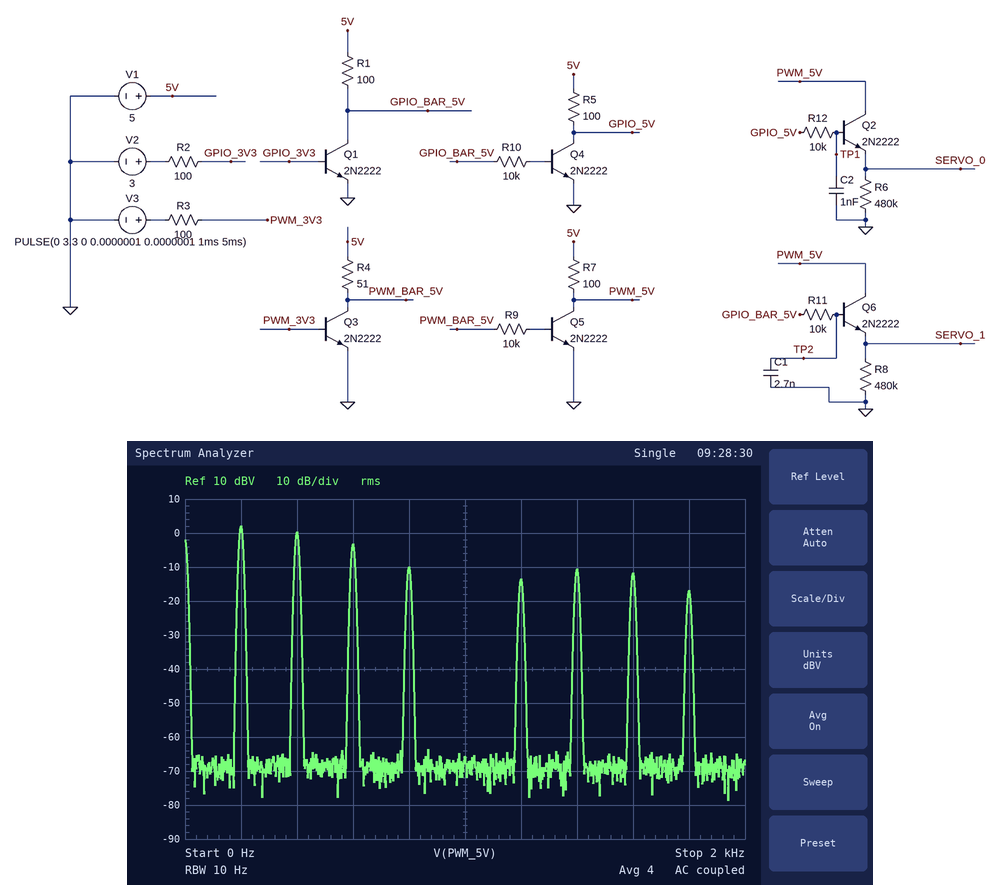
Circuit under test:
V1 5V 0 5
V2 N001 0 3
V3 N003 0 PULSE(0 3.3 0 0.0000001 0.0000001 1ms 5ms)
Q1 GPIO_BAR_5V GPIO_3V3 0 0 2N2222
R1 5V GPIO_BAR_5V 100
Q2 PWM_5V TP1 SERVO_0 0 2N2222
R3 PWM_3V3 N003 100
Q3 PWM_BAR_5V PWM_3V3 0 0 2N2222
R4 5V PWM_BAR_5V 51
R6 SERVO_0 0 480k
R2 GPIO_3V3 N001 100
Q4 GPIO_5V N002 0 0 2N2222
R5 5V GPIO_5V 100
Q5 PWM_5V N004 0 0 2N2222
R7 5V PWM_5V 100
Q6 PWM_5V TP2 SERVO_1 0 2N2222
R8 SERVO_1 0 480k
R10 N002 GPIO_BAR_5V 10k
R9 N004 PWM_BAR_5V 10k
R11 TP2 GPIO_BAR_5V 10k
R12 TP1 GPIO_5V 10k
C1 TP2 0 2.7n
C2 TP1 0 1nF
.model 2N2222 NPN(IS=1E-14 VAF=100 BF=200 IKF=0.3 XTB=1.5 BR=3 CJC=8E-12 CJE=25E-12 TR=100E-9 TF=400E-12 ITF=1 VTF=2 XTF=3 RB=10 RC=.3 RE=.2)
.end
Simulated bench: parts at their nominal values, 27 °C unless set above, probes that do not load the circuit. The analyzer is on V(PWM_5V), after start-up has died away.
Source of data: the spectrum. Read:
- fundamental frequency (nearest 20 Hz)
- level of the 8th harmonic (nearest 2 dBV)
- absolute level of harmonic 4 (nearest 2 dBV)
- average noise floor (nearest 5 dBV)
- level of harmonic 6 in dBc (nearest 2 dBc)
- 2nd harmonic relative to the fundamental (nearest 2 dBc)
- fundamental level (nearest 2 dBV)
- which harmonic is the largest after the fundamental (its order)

200 Hz
-12 dBV
-10 dBV
-70 dBV
-16 dBc
-2 dBc
2 dBV
2
